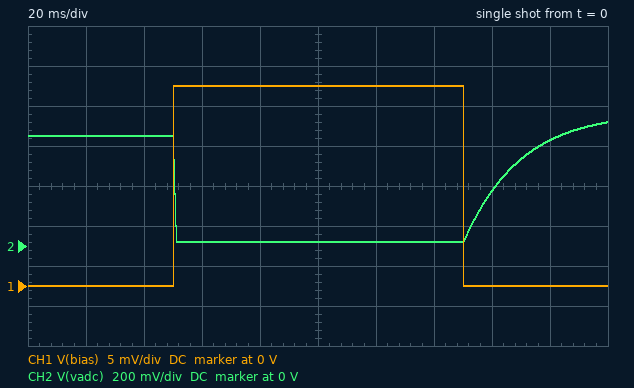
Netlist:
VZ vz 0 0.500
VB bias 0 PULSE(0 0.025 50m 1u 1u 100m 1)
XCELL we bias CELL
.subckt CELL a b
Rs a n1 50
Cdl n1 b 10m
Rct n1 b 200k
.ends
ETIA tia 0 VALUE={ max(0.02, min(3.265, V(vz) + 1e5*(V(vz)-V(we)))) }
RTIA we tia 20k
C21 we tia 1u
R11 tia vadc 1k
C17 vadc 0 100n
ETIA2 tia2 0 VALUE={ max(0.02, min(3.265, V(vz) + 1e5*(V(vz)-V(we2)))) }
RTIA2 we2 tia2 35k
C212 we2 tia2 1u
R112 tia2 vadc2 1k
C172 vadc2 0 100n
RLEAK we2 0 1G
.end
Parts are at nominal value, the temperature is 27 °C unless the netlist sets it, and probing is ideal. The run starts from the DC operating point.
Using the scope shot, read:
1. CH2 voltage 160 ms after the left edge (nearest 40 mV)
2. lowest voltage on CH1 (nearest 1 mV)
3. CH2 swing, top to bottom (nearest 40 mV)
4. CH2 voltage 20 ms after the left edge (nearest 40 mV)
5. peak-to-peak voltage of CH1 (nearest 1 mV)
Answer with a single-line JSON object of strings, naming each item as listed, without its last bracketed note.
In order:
{"CH2 voltage 160 ms after the left edge": "280 mV", "lowest voltage on CH1": "0 V", "CH2 swing, top to bottom": "600 mV", "CH2 voltage 20 ms after the left edge": "560 mV", "peak-to-peak voltage of CH1": "25 mV"}
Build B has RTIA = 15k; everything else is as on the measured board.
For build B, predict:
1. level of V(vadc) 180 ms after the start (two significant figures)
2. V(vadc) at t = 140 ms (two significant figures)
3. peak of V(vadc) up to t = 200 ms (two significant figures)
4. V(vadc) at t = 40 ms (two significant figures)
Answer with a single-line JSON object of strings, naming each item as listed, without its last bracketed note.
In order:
{"level of V(vadc) 180 ms after the start": "570 mV", "V(vadc) at t = 140 ms": "20 mV", "peak of V(vadc) up to t = 200 ms": "630 mV", "V(vadc) at t = 40 ms": "540 mV"}
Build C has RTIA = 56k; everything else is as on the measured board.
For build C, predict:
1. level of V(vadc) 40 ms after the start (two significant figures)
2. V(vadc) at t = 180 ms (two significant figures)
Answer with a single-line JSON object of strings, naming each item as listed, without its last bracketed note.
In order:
{"level of V(vadc) 40 ms after the start": "640 mV", "V(vadc) at t = 180 ms": "360 mV"}
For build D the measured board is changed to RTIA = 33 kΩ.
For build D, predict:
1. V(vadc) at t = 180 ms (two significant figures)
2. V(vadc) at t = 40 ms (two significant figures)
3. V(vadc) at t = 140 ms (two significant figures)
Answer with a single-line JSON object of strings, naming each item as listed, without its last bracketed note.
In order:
{"V(vadc) at t = 180 ms": "440 mV", "V(vadc) at t = 40 ms": "580 mV", "V(vadc) at t = 140 ms": "20 mV"}
